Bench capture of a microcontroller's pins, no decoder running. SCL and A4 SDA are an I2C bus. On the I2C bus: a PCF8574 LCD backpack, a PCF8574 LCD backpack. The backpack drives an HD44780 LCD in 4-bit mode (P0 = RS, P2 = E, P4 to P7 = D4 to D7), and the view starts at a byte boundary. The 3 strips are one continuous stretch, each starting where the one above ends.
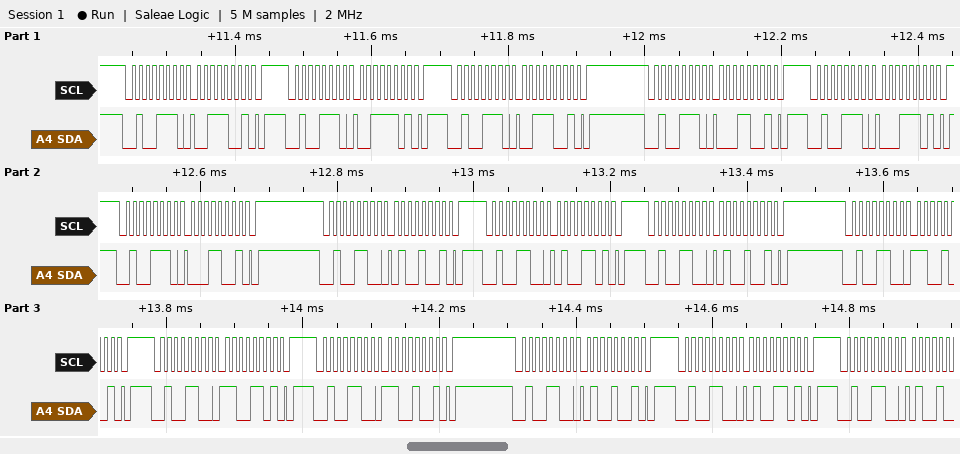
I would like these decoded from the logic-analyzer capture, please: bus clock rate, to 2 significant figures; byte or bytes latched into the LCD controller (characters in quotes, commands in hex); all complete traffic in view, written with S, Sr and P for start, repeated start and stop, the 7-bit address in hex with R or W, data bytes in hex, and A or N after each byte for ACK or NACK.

100 kHz
'1' 'L'
S 27W A 39 A P S 27W A 3D A P S 27W A 39 A P S 27W A 19 A P S 27W A 1D A P S 27W A 19 A P S 26W A 49 A P S 26W A 4D A P S 26W A 49 A P S 26W A C9 A P S 26W A CD A P S 26W A C9 A P S 26W A 49 A P S 26W A 4D A P S 26W A
